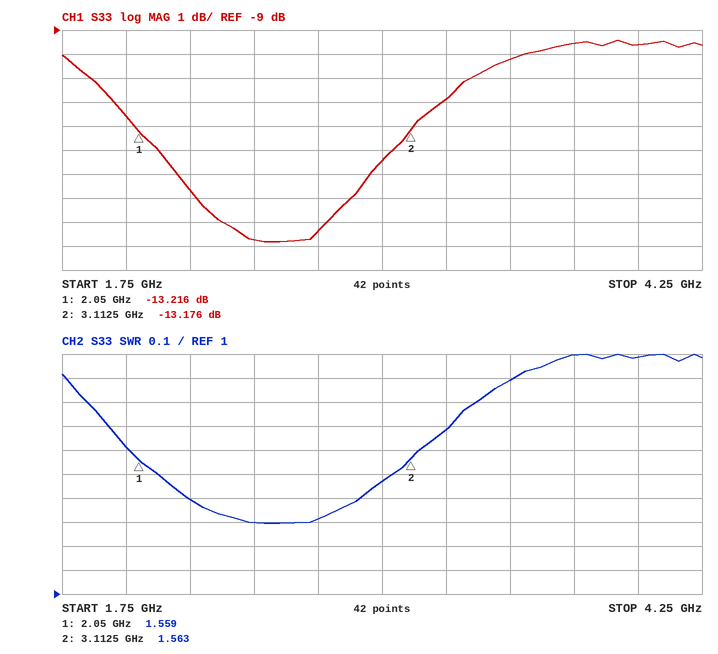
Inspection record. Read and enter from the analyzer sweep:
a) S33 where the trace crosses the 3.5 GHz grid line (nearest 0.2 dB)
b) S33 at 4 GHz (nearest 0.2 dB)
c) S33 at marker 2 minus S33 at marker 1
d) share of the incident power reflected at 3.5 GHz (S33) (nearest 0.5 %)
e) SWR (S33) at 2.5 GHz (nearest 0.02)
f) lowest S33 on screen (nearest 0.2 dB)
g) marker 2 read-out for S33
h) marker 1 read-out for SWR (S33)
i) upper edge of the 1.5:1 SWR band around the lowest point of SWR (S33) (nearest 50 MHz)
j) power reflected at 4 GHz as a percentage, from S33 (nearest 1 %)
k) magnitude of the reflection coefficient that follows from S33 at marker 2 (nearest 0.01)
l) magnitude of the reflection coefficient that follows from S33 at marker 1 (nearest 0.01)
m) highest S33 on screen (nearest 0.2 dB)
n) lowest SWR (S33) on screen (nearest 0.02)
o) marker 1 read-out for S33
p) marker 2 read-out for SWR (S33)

-10.2 dB
-9.6 dB
0.040 dB
9.5 %
1.30
-17.8 dB
-13.176 dB
1.559
3.05 GHz
11 %
0.22
0.22
-9.4 dB
1.30
-13.216 dB
1.563
